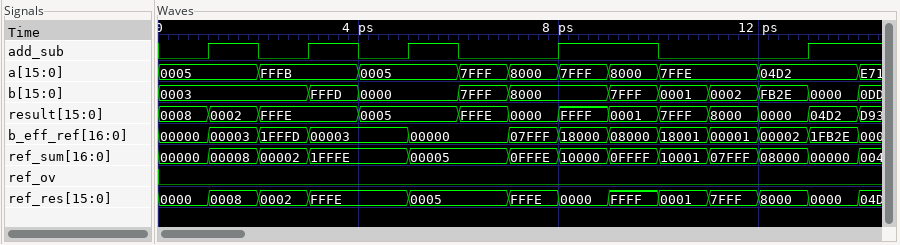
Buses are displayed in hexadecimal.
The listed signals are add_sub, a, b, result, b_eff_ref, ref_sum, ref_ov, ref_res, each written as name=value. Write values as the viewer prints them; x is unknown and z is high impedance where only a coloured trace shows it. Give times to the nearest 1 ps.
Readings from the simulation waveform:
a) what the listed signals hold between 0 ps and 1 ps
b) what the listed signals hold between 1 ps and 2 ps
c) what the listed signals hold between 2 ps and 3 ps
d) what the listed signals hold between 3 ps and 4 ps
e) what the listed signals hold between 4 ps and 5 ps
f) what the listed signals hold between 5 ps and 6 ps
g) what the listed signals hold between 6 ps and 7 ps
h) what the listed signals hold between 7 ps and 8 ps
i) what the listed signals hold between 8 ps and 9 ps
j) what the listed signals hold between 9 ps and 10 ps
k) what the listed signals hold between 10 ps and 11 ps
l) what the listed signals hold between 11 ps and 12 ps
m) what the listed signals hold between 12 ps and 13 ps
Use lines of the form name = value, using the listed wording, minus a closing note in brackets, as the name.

what the listed signals hold between 0 ps and 1 ps = add_sub=0, a=0005, b=0003, result=0008, b_eff_ref=00000, ref_sum=00000, ref_ov=0, ref_res=0000
what the listed signals hold between 1 ps and 2 ps = add_sub=1, a=0005, b=0003, result=0002, b_eff_ref=00003, ref_sum=00008, ref_ov=0, ref_res=0008
what the listed signals hold between 2 ps and 3 ps = add_sub=0, a=FFFB, b=0003, result=FFFE, b_eff_ref=1FFFD, ref_sum=00002, ref_ov=0, ref_res=0002
what the listed signals hold between 3 ps and 4 ps = add_sub=1, a=FFFB, b=FFFD, result=FFFE, b_eff_ref=00003, ref_sum=1FFFE, ref_ov=0, ref_res=FFFE
what the listed signals hold between 4 ps and 5 ps = add_sub=0, a=0005, b=0000, result=0005, b_eff_ref=00003, ref_sum=1FFFE, ref_ov=0, ref_res=FFFE
what the listed signals hold between 5 ps and 6 ps = add_sub=1, a=0005, b=0000, result=0005, b_eff_ref=00000, ref_sum=00005, ref_ov=0, ref_res=0005
what the listed signals hold between 6 ps and 7 ps = add_sub=0, a=7FFF, b=7FFF, result=FFFE, b_eff_ref=00000, ref_sum=00005, ref_ov=0, ref_res=0005
what the listed signals hold between 7 ps and 8 ps = add_sub=0, a=8000, b=8000, result=0000, b_eff_ref=07FFF, ref_sum=0FFFE, ref_ov=0, ref_res=FFFE
what the listed signals hold between 8 ps and 9 ps = add_sub=1, a=7FFF, b=8000, result=FFFF, b_eff_ref=18000, ref_sum=10000, ref_ov=0, ref_res=0000
what the listed signals hold between 9 ps and 10 ps = add_sub=1, a=8000, b=7FFF, result=0001, b_eff_ref=08000, ref_sum=0FFFF, ref_ov=0, ref_res=FFFF
what the listed signals hold between 10 ps and 11 ps = add_sub=0, a=7FFE, b=0001, result=7FFF, b_eff_ref=18001, ref_sum=10001, ref_ov=0, ref_res=0001
what the listed signals hold between 11 ps and 12 ps = add_sub=0, a=7FFE, b=0002, result=8000, b_eff_ref=00001, ref_sum=07FFF, ref_ov=0, ref_res=7FFF
what the listed signals hold between 12 ps and 13 ps = add_sub=0, a=04D2, b=FB2E, result=0000, b_eff_ref=00002, ref_sum=08000, ref_ov=0, ref_res=8000
